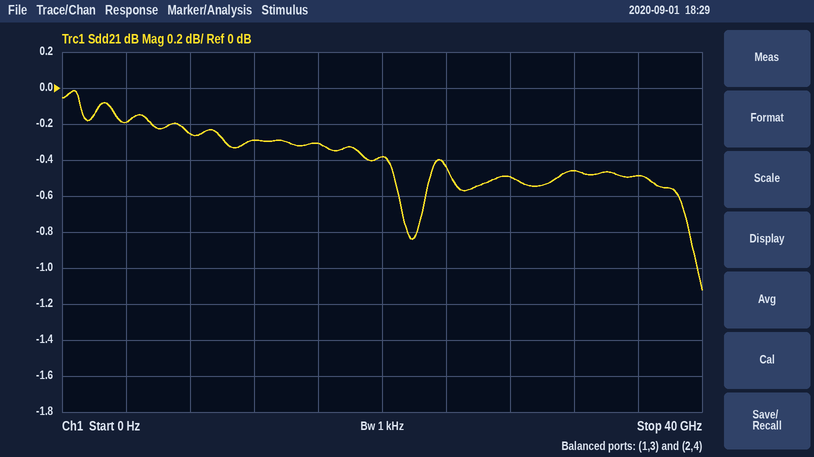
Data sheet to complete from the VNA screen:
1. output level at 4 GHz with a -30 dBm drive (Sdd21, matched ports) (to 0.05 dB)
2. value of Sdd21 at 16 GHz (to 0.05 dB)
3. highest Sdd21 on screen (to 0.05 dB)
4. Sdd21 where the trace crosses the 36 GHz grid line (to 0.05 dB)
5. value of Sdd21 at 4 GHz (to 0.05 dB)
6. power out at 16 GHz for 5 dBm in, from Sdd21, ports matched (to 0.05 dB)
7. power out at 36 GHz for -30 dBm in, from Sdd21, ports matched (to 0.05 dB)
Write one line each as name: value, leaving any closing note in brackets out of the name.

output level at 4 GHz with a -30 dBm drive (Sdd21, matched ports): -30.20 dBm
value of Sdd21 at 16 GHz: -0.30 dB
highest Sdd21 on screen: 0.00 dB
Sdd21 where the trace crosses the 36 GHz grid line: -0.50 dB
value of Sdd21 at 4 GHz: -0.20 dB
power out at 16 GHz for 5 dBm in, from Sdd21, ports matched: 4.70 dBm
power out at 36 GHz for -30 dBm in, from Sdd21, ports matched: -30.50 dBm
